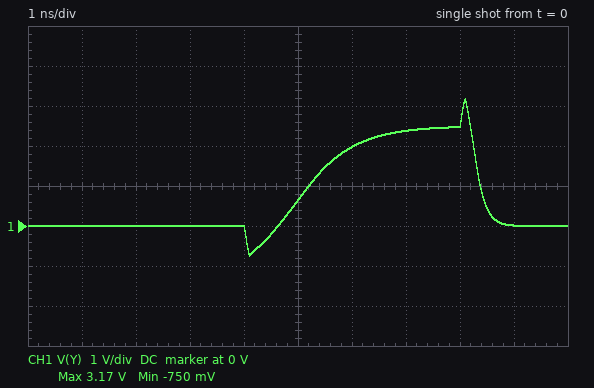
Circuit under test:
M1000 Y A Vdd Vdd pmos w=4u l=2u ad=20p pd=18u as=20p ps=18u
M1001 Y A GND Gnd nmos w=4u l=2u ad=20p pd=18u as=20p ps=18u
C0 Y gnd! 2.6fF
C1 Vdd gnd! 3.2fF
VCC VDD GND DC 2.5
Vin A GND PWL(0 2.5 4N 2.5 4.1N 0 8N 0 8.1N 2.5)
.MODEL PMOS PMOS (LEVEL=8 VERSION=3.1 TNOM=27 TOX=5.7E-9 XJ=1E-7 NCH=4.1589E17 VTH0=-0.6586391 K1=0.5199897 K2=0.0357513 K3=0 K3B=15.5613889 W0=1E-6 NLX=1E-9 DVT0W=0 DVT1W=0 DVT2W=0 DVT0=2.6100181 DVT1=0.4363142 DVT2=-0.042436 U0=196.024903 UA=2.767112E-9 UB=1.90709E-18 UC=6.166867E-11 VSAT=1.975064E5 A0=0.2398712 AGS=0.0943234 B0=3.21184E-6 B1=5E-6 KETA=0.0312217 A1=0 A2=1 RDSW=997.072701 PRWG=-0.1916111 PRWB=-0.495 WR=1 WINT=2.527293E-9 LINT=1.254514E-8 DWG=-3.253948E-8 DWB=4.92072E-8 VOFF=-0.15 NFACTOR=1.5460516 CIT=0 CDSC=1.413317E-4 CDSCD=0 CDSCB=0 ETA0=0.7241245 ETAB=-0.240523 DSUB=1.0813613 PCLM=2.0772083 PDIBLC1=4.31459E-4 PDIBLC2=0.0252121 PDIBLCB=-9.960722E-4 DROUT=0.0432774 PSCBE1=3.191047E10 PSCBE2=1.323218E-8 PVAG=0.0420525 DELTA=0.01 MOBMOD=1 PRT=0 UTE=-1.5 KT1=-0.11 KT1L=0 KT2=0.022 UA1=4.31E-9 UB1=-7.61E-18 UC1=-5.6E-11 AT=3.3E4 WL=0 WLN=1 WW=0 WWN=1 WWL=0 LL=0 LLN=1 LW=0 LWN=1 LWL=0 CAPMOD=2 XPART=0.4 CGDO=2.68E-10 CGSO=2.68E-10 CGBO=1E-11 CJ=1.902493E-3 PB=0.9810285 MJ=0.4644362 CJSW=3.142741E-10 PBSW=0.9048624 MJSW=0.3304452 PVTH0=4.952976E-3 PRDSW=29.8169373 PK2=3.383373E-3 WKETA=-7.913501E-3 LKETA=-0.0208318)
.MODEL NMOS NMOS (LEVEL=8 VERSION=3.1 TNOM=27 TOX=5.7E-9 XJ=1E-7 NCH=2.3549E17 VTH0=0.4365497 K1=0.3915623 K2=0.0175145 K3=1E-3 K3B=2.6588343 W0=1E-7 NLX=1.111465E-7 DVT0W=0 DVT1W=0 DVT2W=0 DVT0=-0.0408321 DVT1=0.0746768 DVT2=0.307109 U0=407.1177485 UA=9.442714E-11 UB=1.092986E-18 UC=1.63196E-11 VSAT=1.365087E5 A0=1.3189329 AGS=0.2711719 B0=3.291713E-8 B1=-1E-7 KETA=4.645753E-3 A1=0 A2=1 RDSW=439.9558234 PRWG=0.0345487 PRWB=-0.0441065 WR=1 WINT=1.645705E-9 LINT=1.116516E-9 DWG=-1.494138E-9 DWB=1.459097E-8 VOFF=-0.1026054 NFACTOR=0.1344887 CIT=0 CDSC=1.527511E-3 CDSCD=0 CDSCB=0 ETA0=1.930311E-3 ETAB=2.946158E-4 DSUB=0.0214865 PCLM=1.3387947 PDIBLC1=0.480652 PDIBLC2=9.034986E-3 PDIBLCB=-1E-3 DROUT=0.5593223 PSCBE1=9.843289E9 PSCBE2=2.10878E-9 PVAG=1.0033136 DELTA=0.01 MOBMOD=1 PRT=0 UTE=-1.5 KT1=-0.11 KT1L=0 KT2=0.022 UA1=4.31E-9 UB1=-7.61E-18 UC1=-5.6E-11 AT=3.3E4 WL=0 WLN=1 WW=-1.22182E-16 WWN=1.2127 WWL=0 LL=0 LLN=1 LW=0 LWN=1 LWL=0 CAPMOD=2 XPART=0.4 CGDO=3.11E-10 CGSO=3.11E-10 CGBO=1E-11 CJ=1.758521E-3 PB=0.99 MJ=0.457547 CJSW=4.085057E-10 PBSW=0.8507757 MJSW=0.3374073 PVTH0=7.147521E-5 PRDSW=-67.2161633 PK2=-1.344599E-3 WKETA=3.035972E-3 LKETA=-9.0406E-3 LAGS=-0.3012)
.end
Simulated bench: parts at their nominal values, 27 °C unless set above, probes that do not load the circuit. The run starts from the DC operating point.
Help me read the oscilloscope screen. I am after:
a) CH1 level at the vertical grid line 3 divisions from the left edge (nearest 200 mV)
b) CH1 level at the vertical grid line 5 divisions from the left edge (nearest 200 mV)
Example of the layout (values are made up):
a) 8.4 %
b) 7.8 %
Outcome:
a) 0 V
b) 600 mV
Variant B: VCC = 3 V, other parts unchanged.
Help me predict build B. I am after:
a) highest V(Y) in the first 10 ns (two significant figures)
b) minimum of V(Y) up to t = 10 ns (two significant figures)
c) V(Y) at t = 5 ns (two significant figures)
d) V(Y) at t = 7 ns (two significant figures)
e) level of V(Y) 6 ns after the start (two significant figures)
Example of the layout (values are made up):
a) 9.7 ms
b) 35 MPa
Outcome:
a) 3.7 V
b) -780 mV
c) 1.3 V
d) 2.9 V
e) 2.7 V
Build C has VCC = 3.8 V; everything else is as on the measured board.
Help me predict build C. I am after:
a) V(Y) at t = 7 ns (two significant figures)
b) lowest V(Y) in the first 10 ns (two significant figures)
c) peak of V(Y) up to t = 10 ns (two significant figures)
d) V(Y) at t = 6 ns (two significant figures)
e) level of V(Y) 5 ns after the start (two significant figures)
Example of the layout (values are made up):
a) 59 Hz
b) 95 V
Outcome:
a) 3.8 V
b) -730 mV
c) 4.5 V
d) 3.6 V
e) 2.4 V
